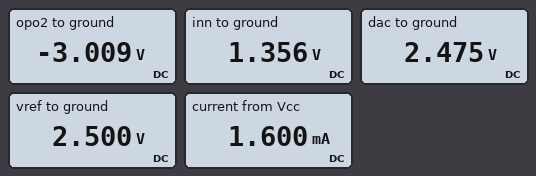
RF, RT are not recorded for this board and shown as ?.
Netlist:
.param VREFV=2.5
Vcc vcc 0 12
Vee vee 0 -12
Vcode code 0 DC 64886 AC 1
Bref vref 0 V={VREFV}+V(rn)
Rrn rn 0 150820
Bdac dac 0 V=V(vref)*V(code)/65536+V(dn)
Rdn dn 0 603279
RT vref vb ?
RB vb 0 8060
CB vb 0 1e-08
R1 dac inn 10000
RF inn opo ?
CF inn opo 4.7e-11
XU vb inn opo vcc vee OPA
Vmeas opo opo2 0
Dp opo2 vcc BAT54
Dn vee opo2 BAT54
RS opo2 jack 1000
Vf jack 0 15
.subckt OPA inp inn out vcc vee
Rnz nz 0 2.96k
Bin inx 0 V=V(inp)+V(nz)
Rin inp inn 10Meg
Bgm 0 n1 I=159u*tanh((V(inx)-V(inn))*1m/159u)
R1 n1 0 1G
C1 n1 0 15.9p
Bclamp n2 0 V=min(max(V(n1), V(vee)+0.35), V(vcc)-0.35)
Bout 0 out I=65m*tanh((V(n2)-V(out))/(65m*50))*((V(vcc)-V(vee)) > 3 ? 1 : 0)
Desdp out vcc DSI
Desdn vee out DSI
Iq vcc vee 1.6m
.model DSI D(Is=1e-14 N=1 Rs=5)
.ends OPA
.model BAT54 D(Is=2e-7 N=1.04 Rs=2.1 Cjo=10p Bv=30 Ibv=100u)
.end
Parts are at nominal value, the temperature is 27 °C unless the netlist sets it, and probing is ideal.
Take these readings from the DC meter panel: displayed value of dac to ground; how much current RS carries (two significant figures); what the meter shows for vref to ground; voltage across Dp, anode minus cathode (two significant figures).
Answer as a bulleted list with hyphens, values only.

- 2.475 V
- 18 mA
- 2.500 V
- -15 V
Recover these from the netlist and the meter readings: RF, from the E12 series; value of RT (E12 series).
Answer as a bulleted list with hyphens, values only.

- 39 kΩ
- 6.8 kΩ
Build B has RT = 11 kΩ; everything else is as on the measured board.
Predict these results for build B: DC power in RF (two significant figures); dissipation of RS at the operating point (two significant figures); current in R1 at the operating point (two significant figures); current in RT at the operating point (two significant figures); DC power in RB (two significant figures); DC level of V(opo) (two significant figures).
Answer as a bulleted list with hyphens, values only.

- 780 µW
- 380 mW
- 140 µA
- 130 µA
- 140 µW
- -4.5 V
